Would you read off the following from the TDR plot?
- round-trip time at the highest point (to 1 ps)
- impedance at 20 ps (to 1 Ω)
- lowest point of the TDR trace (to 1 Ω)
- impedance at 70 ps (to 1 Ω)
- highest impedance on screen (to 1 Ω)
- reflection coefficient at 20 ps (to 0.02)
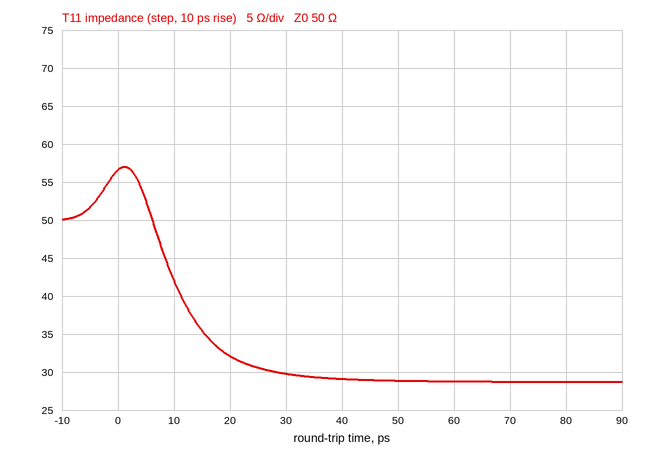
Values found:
1 ps
32 Ω
29 Ω
29 Ω
57 Ω
-0.22
